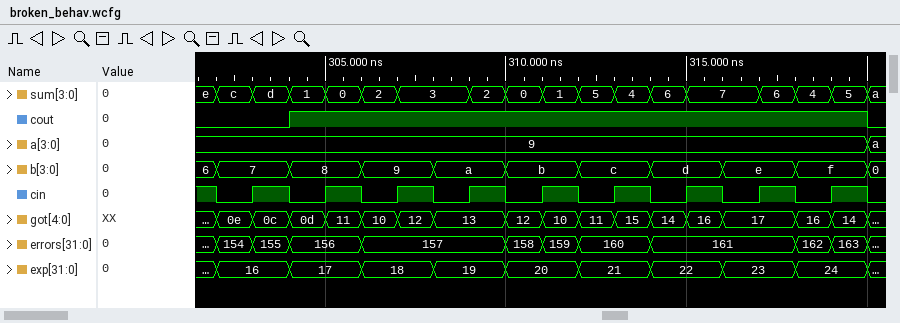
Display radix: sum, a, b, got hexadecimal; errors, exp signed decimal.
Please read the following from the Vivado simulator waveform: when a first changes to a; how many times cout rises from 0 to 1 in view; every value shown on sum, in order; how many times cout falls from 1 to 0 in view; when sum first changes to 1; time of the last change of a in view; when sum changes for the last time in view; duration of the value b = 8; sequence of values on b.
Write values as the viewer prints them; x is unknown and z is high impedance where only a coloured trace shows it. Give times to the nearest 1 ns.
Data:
320 ns
1
e, c, d, 1, 0, 2, 3, 2, 0, 1, 5, 4, 6, 7, 6, 4, 5, a
1
304 ns
320 ns
320 ns
2 ns
6, 7, 8, 9, a, b, c, d, e, f, 0
